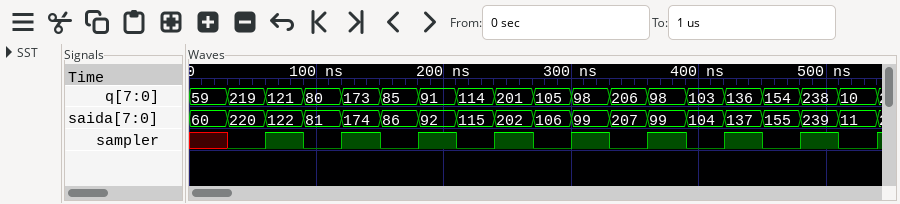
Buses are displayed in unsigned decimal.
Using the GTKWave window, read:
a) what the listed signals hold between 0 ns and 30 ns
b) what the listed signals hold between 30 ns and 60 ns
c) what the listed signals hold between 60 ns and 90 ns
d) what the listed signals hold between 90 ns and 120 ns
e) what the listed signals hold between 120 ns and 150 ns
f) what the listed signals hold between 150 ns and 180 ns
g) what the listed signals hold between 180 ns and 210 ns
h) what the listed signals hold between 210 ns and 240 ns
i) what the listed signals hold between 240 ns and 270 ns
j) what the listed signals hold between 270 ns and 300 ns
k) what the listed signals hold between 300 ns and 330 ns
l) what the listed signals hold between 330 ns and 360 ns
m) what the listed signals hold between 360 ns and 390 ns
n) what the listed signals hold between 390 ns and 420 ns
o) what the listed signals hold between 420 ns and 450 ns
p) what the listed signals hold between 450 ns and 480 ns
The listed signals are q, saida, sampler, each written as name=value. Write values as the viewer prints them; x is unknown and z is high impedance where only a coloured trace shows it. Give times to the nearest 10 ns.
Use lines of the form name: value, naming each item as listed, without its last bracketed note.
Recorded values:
what the listed signals hold between 0 ns and 30 ns: q=59, saida=60, sampler=x
what the listed signals hold between 30 ns and 60 ns: q=219, saida=220, sampler=0
what the listed signals hold between 60 ns and 90 ns: q=121, saida=122, sampler=1
what the listed signals hold between 90 ns and 120 ns: q=80, saida=81, sampler=0
what the listed signals hold between 120 ns and 150 ns: q=173, saida=174, sampler=1
what the listed signals hold between 150 ns and 180 ns: q=85, saida=86, sampler=0
what the listed signals hold between 180 ns and 210 ns: q=91, saida=92, sampler=1
what the listed signals hold between 210 ns and 240 ns: q=114, saida=115, sampler=0
what the listed signals hold between 240 ns and 270 ns: q=201, saida=202, sampler=1
what the listed signals hold between 270 ns and 300 ns: q=105, saida=106, sampler=0
what the listed signals hold between 300 ns and 330 ns: q=98, saida=99, sampler=1
what the listed signals hold between 330 ns and 360 ns: q=206, saida=207, sampler=0
what the listed signals hold between 360 ns and 390 ns: q=98, saida=99, sampler=1
what the listed signals hold between 390 ns and 420 ns: q=103, saida=104, sampler=0
what the listed signals hold between 420 ns and 450 ns: q=136, saida=137, sampler=1
what the listed signals hold between 450 ns and 480 ns: q=154, saida=155, sampler=0
